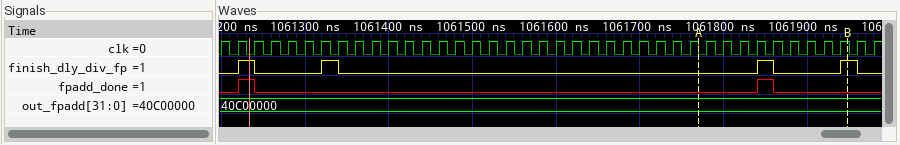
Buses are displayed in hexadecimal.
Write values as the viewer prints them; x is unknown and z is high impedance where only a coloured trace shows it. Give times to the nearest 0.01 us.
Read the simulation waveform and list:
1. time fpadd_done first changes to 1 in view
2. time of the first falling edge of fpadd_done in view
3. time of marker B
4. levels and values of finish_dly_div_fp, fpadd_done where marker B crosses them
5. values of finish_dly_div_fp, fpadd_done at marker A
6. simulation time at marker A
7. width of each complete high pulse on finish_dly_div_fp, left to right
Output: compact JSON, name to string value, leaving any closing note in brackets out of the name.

{"time fpadd_done first changes to 1 in view": "1061.22 us", "time of the first falling edge of fpadd_done in view": "1061.24 us", "time of marker B": "1061.95 us", "levels and values of finish_dly_div_fp, fpadd_done where marker B crosses them": "finish_dly_div_fp=1, fpadd_done=0", "values of finish_dly_div_fp, fpadd_done at marker A": "finish_dly_div_fp=0, fpadd_done=0", "simulation time at marker A": "1061.77 us", "width of each complete high pulse on finish_dly_div_fp, left to right": "0.02 us, 0.02 us, 0.02 us, 0.02 us"}
